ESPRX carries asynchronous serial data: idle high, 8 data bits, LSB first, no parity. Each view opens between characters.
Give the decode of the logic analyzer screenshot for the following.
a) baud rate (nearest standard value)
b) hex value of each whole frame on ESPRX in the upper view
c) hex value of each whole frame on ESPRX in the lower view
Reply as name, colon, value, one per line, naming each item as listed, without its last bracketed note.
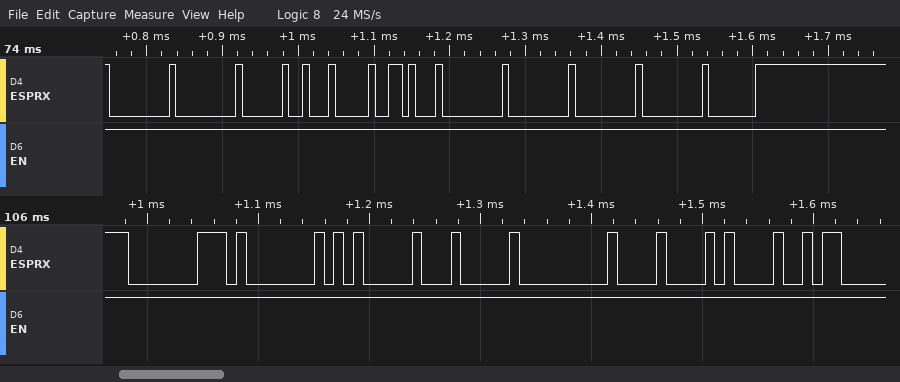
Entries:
baud rate: 115200 baud
hex value of each whole frame on ESPRX in the upper view: 00, 00, 20, 04, 16, 00, 00, 00, 00, C0
hex value of each whole frame on ESPRX in the lower view: C0, 01, 05, 04, 00, 08, 21
